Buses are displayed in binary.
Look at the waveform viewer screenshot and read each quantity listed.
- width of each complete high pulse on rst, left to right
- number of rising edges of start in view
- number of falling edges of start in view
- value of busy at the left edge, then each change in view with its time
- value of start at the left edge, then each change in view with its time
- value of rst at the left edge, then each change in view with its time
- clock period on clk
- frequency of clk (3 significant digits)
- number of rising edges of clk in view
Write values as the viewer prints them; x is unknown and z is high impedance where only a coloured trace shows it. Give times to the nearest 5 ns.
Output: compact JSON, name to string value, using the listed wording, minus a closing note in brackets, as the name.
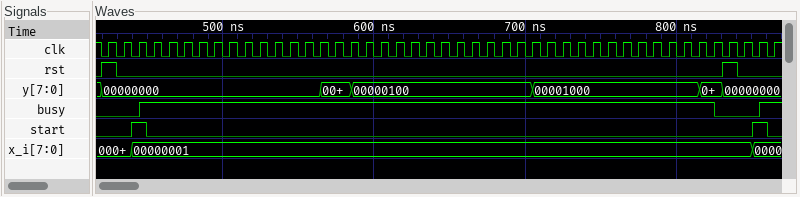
{"width of each complete high pulse on rst, left to right": "10 ns, 10 ns", "number of rising edges of start in view": "2", "number of falling edges of start in view": "2", "value of busy at the left edge, then each change in view with its time": "0, 1 at 445 ns, 0 at 825 ns, 1 at 855 ns", "value of start at the left edge, then each change in view with its time": "0, 1 at 440 ns, 0 at 450 ns, 1 at 850 ns, 0 at 860 ns", "value of rst at the left edge, then each change in view with its time": "0, 1 at 420 ns, 0 at 430 ns, 1 at 830 ns, 0 at 840 ns", "clock period on clk": "10 ns", "frequency of clk": "100 MHz", "number of rising edges of clk in view": "45"}
